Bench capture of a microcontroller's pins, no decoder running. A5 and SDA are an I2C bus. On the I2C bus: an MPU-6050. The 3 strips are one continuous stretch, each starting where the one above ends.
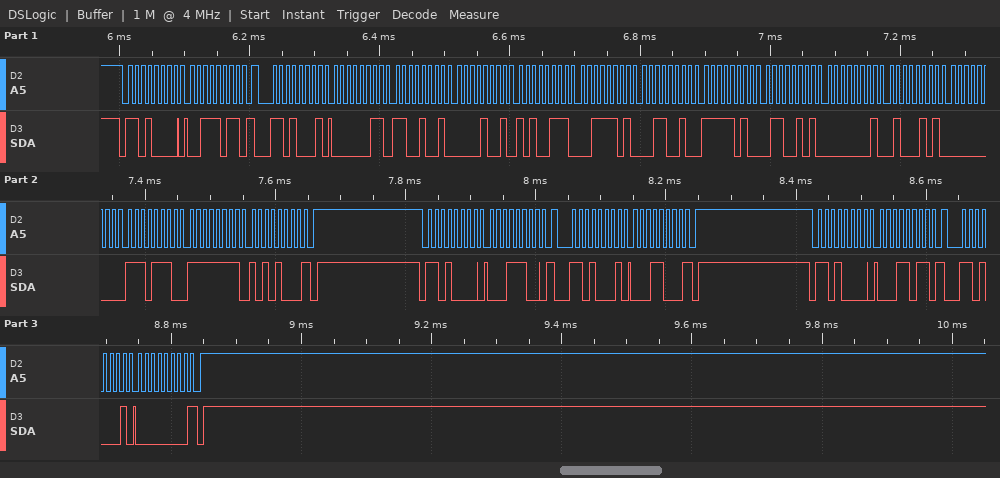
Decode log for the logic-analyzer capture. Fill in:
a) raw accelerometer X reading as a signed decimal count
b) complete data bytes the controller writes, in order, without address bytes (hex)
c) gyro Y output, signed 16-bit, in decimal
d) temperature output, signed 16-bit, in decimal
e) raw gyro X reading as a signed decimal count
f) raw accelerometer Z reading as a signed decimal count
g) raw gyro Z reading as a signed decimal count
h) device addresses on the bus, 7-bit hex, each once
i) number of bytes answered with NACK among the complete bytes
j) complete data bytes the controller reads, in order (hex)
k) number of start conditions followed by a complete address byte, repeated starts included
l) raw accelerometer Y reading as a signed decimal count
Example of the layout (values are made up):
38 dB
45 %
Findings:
969
3B 1C 1B
238
-1435
325
15666
-88
0x68
3
03 C9 09 A7 3D 32 FA 65 01 45 00 EE FF A8 18 00
6
2471
